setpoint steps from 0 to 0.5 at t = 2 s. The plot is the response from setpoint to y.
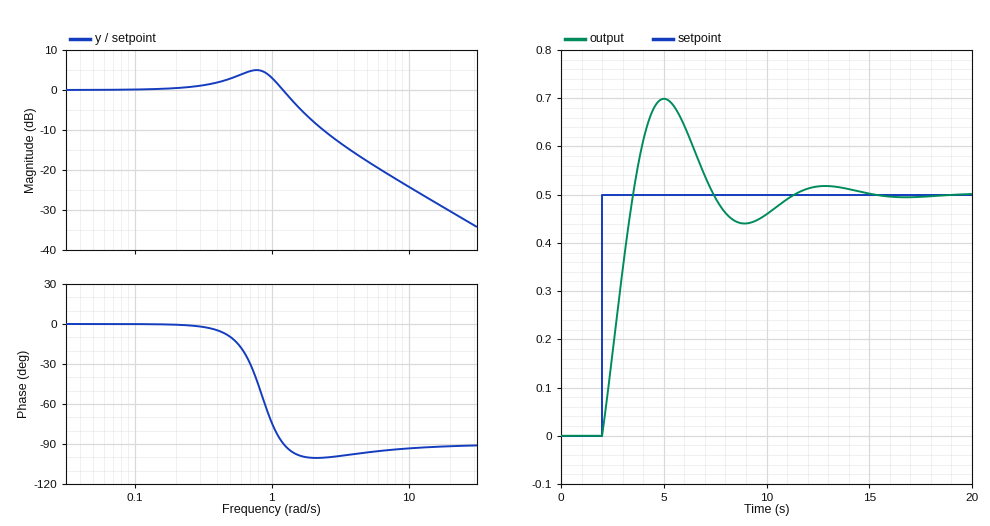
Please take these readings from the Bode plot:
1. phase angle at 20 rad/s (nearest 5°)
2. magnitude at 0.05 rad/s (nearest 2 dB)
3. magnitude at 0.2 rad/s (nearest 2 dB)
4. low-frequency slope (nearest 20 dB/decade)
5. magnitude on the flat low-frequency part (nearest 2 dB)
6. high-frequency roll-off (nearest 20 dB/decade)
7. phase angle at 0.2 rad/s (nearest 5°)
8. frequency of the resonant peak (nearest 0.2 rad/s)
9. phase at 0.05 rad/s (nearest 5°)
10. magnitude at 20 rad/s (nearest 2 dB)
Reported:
-90°
0 dB
0 dB
0 dB/decade
0 dB
-20 dB/decade
0°
0.8 rad/s
0°
-30 dB
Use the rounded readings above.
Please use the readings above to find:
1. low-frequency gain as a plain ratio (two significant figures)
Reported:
1.0
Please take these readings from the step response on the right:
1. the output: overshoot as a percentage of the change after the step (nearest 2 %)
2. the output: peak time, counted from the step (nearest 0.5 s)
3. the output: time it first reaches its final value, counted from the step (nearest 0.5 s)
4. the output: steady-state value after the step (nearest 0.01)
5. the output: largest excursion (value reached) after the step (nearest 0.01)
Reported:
40 %
3.0 s
1.5 s
0.50
0.70
